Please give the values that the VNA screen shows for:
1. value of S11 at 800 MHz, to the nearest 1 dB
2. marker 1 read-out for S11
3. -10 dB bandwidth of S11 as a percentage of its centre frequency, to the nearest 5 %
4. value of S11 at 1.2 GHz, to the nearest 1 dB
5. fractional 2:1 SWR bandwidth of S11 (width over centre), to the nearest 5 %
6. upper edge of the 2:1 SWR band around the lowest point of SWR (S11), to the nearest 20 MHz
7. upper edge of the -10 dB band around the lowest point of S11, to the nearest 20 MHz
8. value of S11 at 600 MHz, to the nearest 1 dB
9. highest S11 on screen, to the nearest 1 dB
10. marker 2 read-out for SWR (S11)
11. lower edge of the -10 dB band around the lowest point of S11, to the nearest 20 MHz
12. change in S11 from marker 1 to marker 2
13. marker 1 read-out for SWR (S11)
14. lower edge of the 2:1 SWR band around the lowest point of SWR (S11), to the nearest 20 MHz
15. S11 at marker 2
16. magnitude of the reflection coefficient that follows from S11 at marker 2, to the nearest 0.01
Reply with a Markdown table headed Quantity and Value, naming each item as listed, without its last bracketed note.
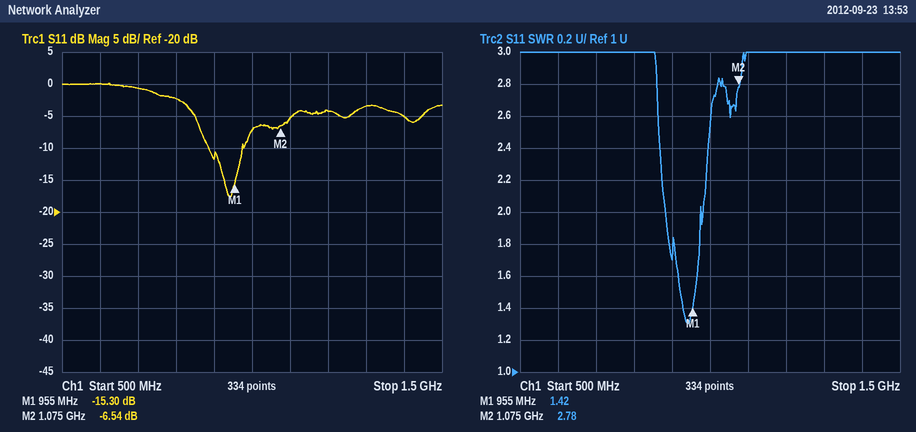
| Quantity | Value |
|---|---|
| value of S11 at 800 MHz, to the nearest 1 dB | -2 dB |
| marker 1 read-out for S11 | -15.30 dB |
| -10 dB bandwidth of S11 as a percentage of its centre frequency, to the nearest 5 % | 10 % |
| value of S11 at 1.2 GHz, to the nearest 1 dB | -4 dB |
| fractional 2:1 SWR bandwidth of S11 (width over centre), to the nearest 5 % | 10 % |
| upper edge of the 2:1 SWR band around the lowest point of SWR (S11), to the nearest 20 MHz | 980 MHz |
| upper edge of the -10 dB band around the lowest point of S11, to the nearest 20 MHz | 980 MHz |
| value of S11 at 600 MHz, to the nearest 1 dB | 0 dB |
| highest S11 on screen, to the nearest 1 dB | 0 dB |
| marker 2 read-out for SWR | 2.78 |
| lower edge of the -10 dB band around the lowest point of S11, to the nearest 20 MHz | 880 MHz |
| change in S11 from marker 1 to marker 2 | 8.76 dB |
| marker 1 read-out for SWR | 1.42 |
| lower edge of the 2:1 SWR band around the lowest point of SWR (S11), to the nearest 20 MHz | 880 MHz |
| S11 at marker 2 | -6.54 dB |
| magnitude of the reflection coefficient that follows from S11 at marker 2, to the nearest 0.01 | 0.47 |
